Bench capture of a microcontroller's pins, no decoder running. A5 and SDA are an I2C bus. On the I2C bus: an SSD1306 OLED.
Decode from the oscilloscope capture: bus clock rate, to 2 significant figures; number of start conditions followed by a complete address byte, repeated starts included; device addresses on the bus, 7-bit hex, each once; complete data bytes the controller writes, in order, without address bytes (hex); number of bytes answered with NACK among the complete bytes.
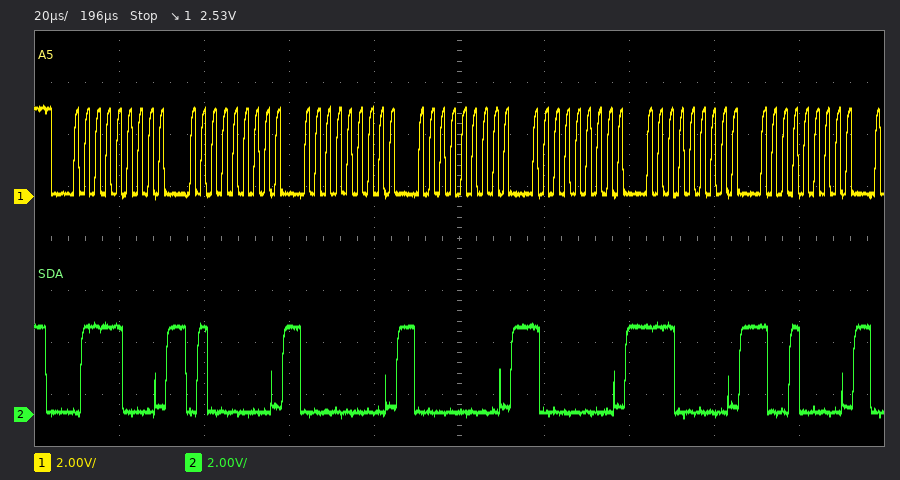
400 kHz
1
0x3C
40 00 00 80 E0 90
0
